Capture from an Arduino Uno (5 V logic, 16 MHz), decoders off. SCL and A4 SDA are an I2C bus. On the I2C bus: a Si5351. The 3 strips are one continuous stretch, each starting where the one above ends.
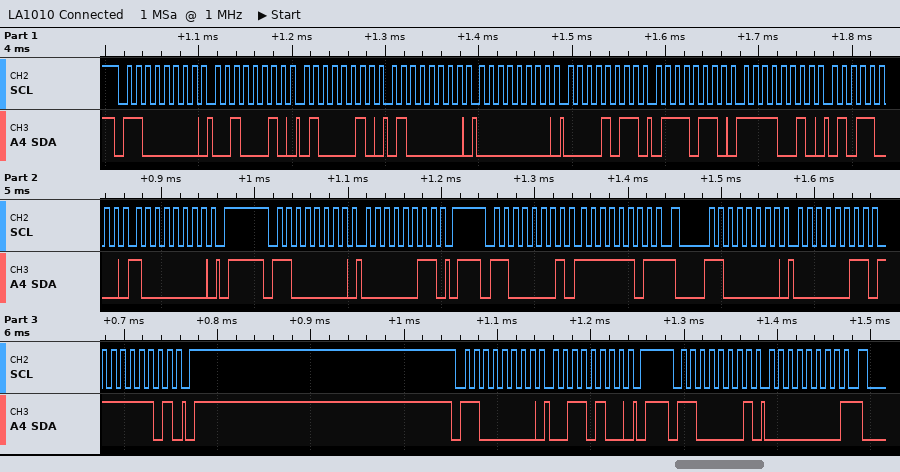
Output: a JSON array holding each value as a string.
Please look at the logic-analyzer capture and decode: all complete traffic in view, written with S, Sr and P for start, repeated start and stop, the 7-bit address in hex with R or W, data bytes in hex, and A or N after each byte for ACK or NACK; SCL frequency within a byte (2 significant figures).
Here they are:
["S 60W A 22 A 42 A 40 A 00 A 0B A 76 A F2 A 58 A 80 A P S 60W A 03 A P S 60R A FD N Sr 60W A 03 A FD A P S 60W A 34 A P S 60R A 00 N", "100 kHz"]
